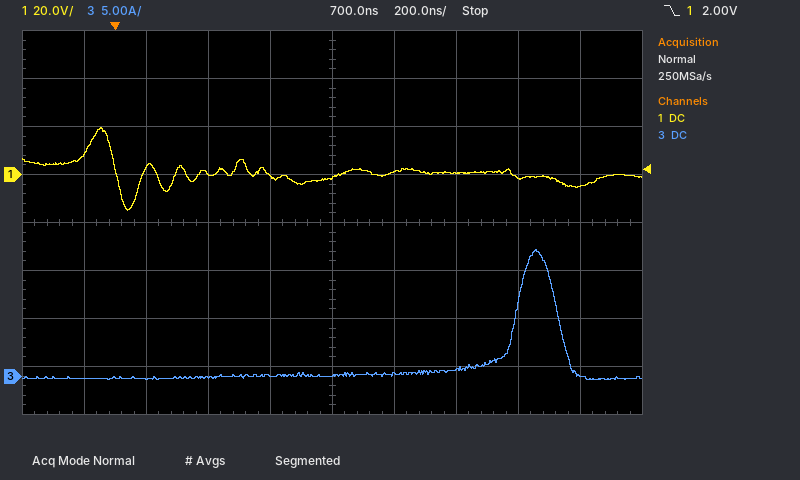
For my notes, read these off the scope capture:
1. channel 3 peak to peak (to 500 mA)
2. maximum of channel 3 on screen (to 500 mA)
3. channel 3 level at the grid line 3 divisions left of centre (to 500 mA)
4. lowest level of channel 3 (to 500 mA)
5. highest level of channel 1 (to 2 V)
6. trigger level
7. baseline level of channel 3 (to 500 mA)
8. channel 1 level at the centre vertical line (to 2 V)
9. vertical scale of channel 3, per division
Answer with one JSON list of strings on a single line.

["13.5 A", "13.0 A", "-500 mA", "-500 mA", "20 V", "2.00 V", "0.0 A", "-2 V", "5 A"]
